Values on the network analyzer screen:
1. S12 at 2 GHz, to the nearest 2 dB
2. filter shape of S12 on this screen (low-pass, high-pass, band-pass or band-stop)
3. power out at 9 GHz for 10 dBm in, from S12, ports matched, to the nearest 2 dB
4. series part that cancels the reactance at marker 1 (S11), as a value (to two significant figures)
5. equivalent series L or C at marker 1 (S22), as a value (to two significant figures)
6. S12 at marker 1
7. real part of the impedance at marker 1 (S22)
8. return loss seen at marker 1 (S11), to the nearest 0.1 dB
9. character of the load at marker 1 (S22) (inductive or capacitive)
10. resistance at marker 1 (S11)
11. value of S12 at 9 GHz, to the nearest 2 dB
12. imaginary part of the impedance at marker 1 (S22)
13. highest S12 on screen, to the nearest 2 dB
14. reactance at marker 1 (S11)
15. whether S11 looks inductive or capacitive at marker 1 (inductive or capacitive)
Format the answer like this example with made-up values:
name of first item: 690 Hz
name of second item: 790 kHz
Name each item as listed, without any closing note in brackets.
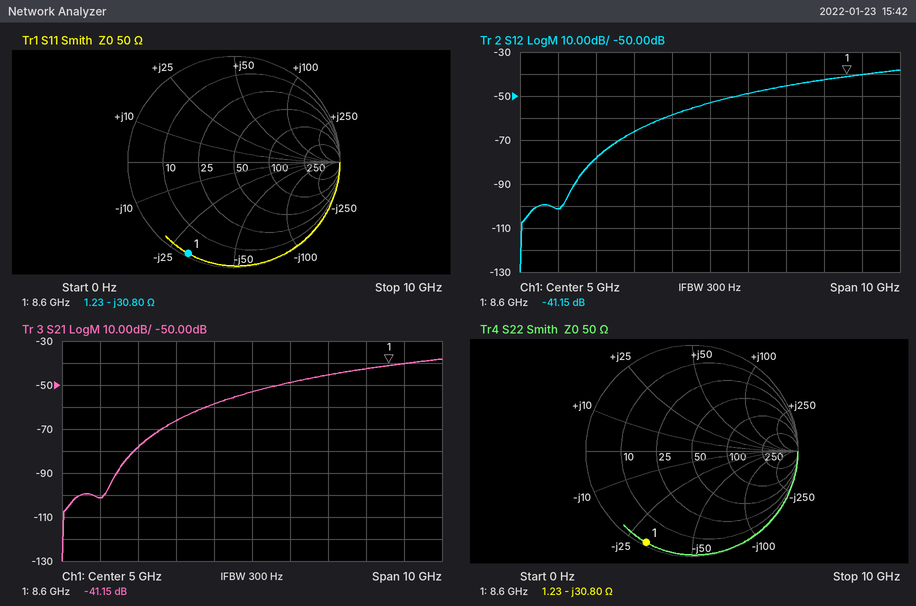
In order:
S12 at 2 GHz, to the nearest 2 dB: -78 dB
filter shape of S12 on this screen: high-pass
power out at 9 GHz for 10 dBm in, from S12, ports matched, to the nearest 2 dB: -30 dBm
series part that cancels the reactance at marker 1 (S11), as a value: 570 pH
equivalent series L or C at marker 1 (S22), as a value: 600 fF
S12 at marker 1: -41.15 dB
real part of the impedance at marker 1: 1.23 Ω
return loss seen at marker 1 (S11), to the nearest 0.1 dB: 0.3 dB
character of the load at marker 1 (S22): capacitive
resistance at marker 1: 1.23 Ω
value of S12 at 9 GHz, to the nearest 2 dB: -40 dB
imaginary part of the impedance at marker 1: -30.80 Ω
highest S12 on screen, to the nearest 2 dB: -38 dB
reactance at marker 1: -30.80 Ω
whether S11 looks inductive or capacitive at marker 1: capacitive
